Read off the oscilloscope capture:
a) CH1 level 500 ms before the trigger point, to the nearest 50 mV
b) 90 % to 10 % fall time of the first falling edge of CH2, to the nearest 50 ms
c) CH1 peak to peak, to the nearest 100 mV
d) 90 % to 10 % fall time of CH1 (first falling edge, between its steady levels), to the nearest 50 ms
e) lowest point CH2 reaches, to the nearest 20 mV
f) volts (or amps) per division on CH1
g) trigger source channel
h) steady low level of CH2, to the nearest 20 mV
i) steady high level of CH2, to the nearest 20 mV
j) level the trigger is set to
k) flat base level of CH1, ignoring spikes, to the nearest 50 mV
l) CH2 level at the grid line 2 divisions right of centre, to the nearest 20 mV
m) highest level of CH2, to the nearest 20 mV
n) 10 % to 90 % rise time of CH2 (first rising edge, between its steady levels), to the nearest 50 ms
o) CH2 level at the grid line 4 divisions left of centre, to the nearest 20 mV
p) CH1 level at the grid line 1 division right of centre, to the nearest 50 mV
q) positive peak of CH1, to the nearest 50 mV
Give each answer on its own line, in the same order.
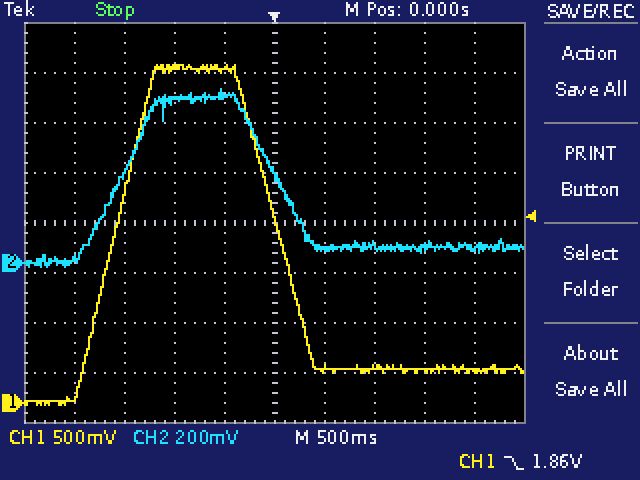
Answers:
3.35 V
600 ms
3.40 V
650 ms
-20 mV
500 mV
CH1
60 mV
660 mV
1.86 V
350 mV
60 mV
700 mV
550 ms
20 mV
350 mV
3.40 V
